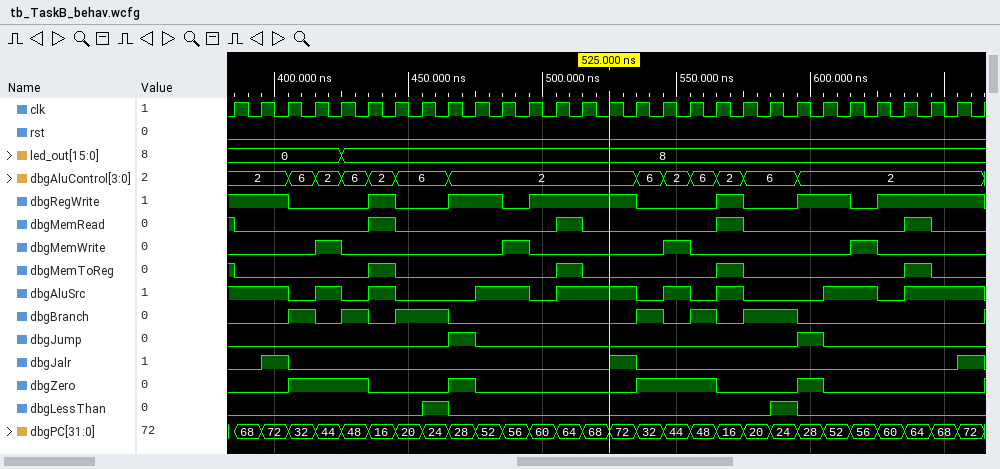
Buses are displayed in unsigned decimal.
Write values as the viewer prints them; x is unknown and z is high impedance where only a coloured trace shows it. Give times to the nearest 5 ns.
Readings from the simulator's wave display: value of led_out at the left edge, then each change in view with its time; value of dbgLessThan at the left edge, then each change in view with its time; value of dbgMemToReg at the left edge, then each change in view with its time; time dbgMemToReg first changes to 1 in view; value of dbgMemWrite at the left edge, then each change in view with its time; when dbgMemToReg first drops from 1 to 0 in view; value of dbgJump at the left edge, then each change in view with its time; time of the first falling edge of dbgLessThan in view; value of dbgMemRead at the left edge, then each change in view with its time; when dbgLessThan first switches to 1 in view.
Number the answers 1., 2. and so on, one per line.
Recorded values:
1. 0, 8 at 425 ns
2. 0, 1 at 455 ns, 0 at 465 ns, 1 at 585 ns, 0 at 595 ns
3. 1, 0 at 385 ns, 1 at 435 ns, 0 at 445 ns, 1 at 505 ns, 0 at 515 ns, 1 at 565 ns, 0 at 575 ns, 1 at 635 ns, 0 at 645 ns
4. 435 ns
5. 0, 1 at 415 ns, 0 at 425 ns, 1 at 485 ns, 0 at 495 ns, 1 at 545 ns, 0 at 555 ns, 1 at 615 ns, 0 at 625 ns
6. 385 ns
7. 0, 1 at 465 ns, 0 at 475 ns, 1 at 595 ns, 0 at 605 ns
8. 465 ns
9. 1, 0 at 385 ns, 1 at 435 ns, 0 at 445 ns, 1 at 505 ns, 0 at 515 ns, 1 at 565 ns, 0 at 575 ns, 1 at 635 ns, 0 at 645 ns
10. 455 ns
